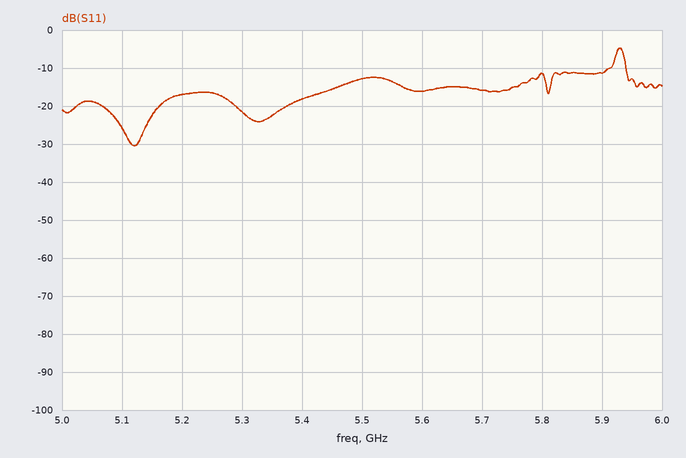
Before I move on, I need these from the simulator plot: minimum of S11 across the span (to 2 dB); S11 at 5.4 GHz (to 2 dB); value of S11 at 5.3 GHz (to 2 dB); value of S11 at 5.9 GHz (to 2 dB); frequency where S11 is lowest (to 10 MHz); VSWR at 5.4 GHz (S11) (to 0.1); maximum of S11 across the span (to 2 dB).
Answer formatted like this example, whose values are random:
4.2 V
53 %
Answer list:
-30 dB
-18 dB
-22 dB
-12 dB
5.12 GHz
1.3
-4 dB
